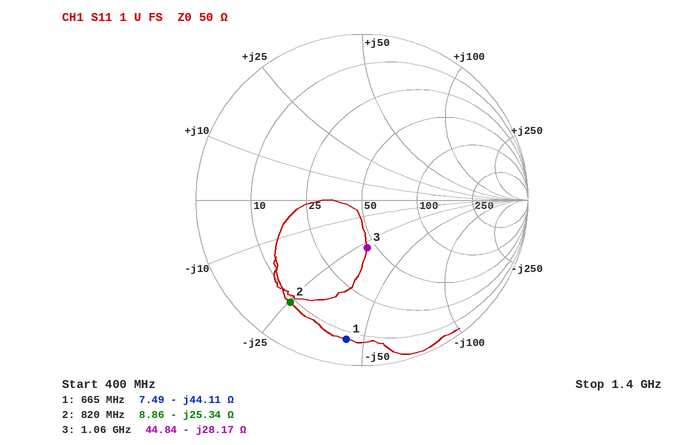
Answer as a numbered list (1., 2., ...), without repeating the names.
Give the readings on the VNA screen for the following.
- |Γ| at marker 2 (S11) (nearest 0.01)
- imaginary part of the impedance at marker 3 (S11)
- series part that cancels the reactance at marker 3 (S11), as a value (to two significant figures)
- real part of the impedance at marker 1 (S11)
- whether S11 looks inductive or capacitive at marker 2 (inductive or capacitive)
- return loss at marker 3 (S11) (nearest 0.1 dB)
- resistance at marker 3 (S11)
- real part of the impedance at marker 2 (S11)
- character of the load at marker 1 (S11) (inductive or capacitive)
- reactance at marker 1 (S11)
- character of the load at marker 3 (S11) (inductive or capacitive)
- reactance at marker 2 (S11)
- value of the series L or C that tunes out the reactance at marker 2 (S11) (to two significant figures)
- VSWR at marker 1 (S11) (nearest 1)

1. 0.75
2. -28.17 Ω
3. 4.2 nH
4. 7.49 Ω
5. capacitive
6. 10.8 dB
7. 44.84 Ω
8. 8.86 Ω
9. capacitive
10. -44.11 Ω
11. capacitive
12. -25.34 Ω
13. 4.9 nH
14. 12
